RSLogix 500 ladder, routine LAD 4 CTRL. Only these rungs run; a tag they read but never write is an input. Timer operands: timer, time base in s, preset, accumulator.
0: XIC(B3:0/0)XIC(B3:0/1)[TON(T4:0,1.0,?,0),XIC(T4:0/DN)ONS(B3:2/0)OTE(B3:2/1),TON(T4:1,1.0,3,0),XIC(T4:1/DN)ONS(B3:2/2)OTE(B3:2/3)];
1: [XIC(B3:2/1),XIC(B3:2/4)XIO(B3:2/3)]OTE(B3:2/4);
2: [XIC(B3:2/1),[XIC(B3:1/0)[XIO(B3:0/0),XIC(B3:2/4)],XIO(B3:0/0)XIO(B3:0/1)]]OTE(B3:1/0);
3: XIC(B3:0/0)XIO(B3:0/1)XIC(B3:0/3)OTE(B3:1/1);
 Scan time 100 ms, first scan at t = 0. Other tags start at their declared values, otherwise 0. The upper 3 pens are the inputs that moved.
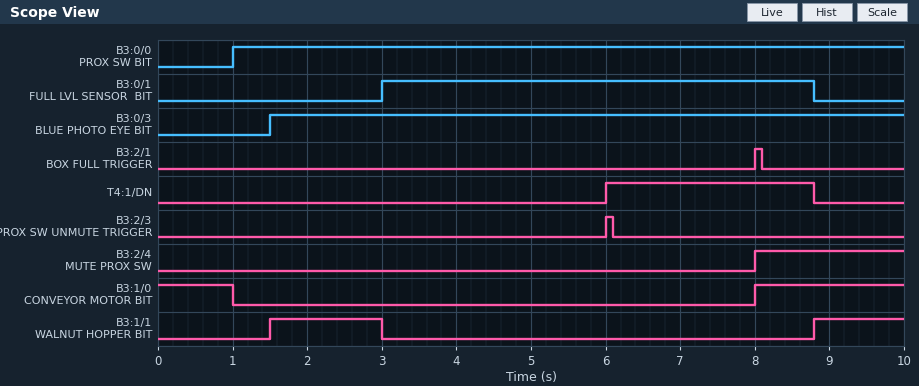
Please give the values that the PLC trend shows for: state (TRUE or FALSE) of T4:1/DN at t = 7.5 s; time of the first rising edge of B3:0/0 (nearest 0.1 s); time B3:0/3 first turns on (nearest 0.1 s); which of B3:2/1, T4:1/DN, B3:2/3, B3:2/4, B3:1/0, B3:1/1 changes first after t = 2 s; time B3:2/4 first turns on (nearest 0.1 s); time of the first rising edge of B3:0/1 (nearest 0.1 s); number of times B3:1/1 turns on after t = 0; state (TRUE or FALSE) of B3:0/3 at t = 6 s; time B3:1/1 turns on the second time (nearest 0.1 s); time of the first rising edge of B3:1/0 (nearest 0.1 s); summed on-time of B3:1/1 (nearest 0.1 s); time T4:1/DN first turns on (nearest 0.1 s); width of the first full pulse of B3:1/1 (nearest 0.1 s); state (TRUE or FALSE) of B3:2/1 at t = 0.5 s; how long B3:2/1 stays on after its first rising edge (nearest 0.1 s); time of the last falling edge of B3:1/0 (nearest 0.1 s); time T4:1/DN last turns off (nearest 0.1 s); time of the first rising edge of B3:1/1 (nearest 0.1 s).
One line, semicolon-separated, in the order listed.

TRUE; 1.0 s; 1.5 s; B3:1/1; 8.0 s; 3.0 s; 2; TRUE; 8.8 s; 8.0 s; 2.7 s; 6.0 s; 1.5 s; FALSE; 0.1 s; 1.0 s; 8.8 s; 1.5 s
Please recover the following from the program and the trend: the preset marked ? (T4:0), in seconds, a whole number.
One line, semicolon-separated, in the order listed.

5 s
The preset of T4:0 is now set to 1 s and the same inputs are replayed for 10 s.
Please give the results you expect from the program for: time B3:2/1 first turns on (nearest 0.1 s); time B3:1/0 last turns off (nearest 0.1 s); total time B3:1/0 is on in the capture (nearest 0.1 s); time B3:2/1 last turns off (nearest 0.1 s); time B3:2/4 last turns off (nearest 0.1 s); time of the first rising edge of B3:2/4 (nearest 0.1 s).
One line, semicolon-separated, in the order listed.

4.0 s; 6.0 s; 3.0 s; 4.1 s; 6.0 s; 4.0 s
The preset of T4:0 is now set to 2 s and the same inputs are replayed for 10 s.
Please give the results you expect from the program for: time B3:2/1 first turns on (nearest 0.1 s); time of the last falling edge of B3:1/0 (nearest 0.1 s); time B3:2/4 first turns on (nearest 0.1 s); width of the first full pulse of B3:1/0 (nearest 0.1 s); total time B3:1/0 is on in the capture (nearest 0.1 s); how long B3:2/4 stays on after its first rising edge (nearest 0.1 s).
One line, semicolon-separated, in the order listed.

5.0 s; 6.0 s; 5.0 s; 1.0 s; 2.0 s; 1.0 s
